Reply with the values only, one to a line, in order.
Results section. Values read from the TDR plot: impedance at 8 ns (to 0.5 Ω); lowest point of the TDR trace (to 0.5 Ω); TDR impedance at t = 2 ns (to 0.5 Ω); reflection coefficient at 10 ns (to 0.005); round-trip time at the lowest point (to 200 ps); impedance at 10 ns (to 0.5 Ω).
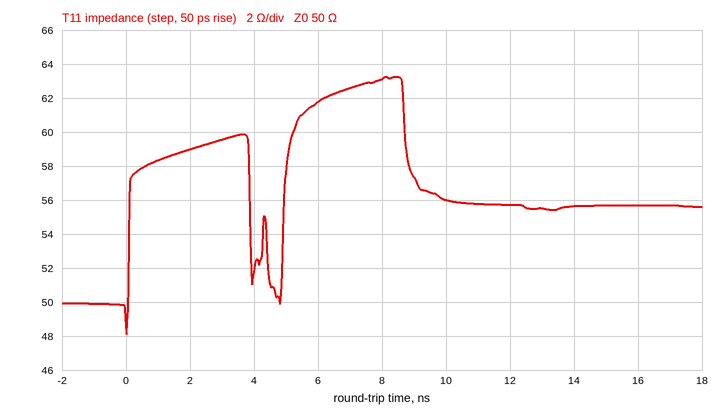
63.0 Ω
48.0 Ω
59.0 Ω
+0.055
0.0 ns
56.0 Ω
